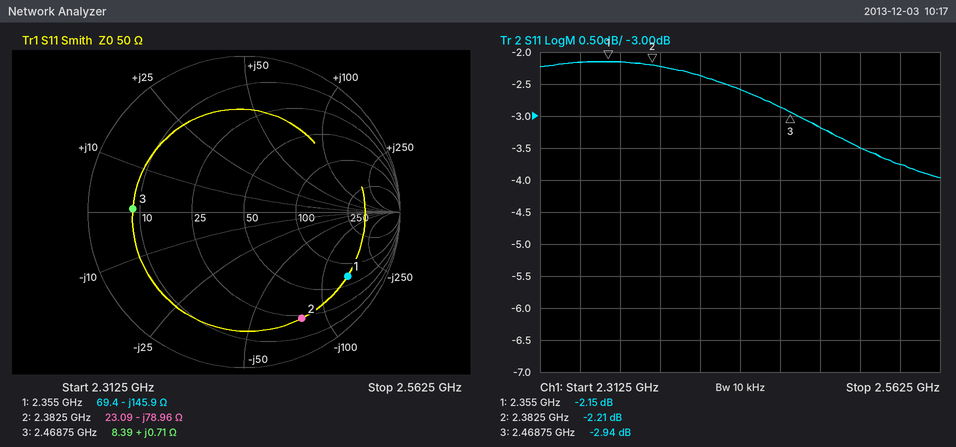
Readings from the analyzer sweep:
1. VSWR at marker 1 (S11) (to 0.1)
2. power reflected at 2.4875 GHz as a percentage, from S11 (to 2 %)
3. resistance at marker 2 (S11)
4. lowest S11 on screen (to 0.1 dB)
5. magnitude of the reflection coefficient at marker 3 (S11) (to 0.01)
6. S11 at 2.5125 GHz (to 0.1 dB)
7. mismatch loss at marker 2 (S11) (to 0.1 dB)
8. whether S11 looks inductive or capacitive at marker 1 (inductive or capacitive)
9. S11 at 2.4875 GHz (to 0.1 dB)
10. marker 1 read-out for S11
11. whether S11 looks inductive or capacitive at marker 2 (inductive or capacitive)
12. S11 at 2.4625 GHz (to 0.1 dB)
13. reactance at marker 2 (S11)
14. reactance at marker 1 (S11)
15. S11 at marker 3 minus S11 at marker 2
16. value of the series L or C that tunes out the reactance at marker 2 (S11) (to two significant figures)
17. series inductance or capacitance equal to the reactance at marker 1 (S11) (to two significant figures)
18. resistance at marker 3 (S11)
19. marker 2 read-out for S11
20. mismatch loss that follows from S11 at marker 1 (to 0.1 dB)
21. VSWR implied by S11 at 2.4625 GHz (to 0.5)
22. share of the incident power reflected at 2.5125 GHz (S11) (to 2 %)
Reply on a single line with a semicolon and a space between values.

8.1; 48 %; 23.09 Ω; -4.0 dB; 0.71; -3.5 dB; 4.0 dB; capacitive; -3.2 dB; -2.15 dB; capacitive; -2.9 dB; -78.96 Ω; -145.9 Ω; -0.73 dB; 5.3 nH; 460 fF; 8.39 Ω; -2.21 dB; 4.1 dB; 6.0; 44 %
